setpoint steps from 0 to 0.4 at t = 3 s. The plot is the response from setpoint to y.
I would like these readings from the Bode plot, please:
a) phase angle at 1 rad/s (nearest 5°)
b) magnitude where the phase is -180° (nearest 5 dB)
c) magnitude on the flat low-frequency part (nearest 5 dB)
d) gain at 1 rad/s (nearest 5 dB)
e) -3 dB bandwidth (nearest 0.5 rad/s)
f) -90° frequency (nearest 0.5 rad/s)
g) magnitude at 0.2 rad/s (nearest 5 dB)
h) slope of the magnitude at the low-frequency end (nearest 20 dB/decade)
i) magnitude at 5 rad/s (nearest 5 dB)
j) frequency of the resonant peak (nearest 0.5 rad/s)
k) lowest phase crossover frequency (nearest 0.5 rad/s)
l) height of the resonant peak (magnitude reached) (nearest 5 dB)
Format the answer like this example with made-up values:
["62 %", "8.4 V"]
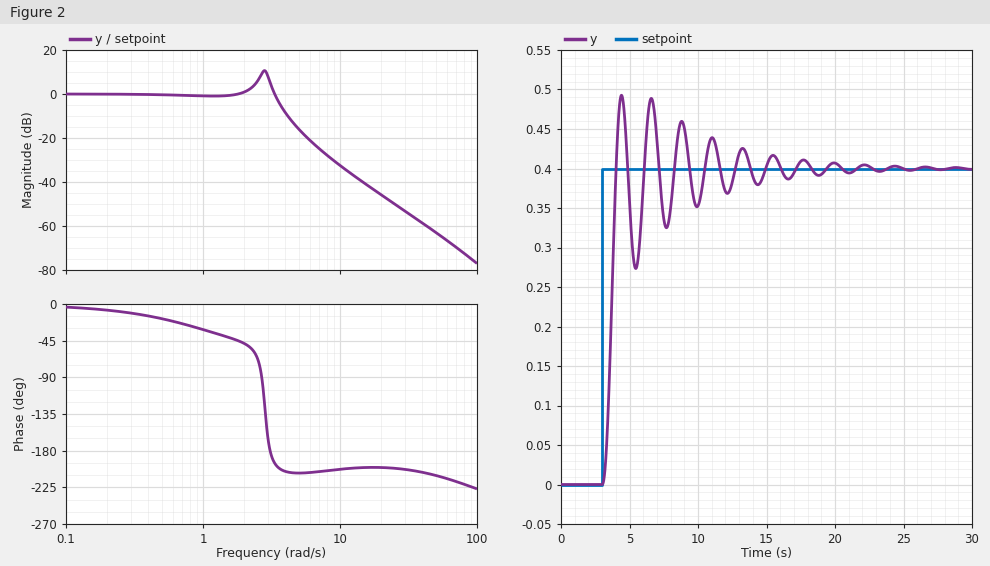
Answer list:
["-30°", "5 dB", "0 dB", "0 dB", "3.5 rad/s", "2.5 rad/s", "0 dB", "0 dB/decade", "-15 dB", "3.0 rad/s", "3.0 rad/s", "10 dB"]
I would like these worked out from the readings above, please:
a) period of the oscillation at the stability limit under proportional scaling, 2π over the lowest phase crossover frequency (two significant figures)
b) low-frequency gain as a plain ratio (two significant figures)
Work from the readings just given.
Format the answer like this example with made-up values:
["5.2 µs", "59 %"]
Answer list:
["2.1 s", "1.0"]
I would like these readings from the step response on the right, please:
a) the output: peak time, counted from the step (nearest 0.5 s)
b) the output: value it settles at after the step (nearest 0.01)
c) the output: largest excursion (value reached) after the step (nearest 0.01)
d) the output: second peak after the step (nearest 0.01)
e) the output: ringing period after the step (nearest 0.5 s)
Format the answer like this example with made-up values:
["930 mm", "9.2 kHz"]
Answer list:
["1.5 s", "0.40", "0.49", "0.49", "2.0 s"]
